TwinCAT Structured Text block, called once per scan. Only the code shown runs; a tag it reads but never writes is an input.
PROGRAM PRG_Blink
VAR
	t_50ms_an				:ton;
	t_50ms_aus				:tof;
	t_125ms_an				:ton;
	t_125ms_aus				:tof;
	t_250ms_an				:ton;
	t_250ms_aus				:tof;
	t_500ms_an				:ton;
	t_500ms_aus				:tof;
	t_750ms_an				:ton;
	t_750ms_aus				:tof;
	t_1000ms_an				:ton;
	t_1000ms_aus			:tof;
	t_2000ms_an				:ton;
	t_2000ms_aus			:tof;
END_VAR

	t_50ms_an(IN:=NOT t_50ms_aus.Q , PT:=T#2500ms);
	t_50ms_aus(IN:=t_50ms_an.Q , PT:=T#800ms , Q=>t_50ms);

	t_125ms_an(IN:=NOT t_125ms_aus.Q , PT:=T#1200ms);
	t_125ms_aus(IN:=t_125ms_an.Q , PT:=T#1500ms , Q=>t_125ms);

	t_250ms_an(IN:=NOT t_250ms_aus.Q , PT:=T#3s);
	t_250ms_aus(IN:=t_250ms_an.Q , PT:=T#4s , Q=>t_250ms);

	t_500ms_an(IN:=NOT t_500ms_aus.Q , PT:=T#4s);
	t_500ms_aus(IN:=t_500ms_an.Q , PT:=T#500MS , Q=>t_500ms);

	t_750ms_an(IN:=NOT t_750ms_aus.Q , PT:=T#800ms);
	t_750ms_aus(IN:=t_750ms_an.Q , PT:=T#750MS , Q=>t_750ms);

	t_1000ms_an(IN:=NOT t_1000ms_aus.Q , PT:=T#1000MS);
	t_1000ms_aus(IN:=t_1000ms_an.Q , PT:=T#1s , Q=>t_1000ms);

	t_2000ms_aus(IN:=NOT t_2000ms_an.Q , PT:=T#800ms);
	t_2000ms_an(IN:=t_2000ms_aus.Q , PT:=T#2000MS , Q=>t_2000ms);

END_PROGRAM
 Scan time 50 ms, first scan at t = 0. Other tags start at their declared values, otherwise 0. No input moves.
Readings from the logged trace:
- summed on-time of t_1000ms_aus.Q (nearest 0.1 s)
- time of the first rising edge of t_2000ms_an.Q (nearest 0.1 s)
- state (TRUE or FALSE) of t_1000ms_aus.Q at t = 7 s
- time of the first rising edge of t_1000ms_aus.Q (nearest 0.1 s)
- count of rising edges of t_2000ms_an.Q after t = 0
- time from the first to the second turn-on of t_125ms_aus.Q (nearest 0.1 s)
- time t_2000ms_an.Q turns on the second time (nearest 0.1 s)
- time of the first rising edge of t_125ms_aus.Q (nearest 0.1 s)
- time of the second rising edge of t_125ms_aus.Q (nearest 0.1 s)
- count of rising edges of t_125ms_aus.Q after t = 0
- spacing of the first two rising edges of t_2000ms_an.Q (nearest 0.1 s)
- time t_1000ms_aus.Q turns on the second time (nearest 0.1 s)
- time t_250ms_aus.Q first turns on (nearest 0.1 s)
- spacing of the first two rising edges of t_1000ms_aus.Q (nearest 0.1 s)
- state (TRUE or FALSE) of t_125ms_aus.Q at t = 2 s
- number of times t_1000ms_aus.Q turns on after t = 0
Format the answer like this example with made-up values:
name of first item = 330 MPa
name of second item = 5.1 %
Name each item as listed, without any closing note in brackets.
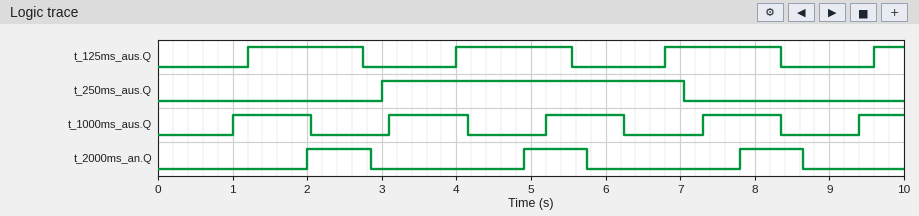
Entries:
summed on-time of t_1000ms_aus.Q = 4.8 s
time of the first rising edge of t_2000ms_an.Q = 2.0 s
state (TRUE or FALSE) of t_1000ms_aus.Q at t = 7 s = FALSE
time of the first rising edge of t_1000ms_aus.Q = 1.0 s
count of rising edges of t_2000ms_an.Q after t = 0 = 3
time from the first to the second turn-on of t_125ms_aus.Q = 2.8 s
time t_2000ms_an.Q turns on the second time = 4.9 s
time of the first rising edge of t_125ms_aus.Q = 1.2 s
time of the second rising edge of t_125ms_aus.Q = 4.0 s
count of rising edges of t_125ms_aus.Q after t = 0 = 4
spacing of the first two rising edges of t_2000ms_an.Q = 2.9 s
time t_1000ms_aus.Q turns on the second time = 3.1 s
time t_250ms_aus.Q first turns on = 3.0 s
spacing of the first two rising edges of t_1000ms_aus.Q = 2.1 s
state (TRUE or FALSE) of t_125ms_aus.Q at t = 2 s = TRUE
number of times t_1000ms_aus.Q turns on after t = 0 = 5
